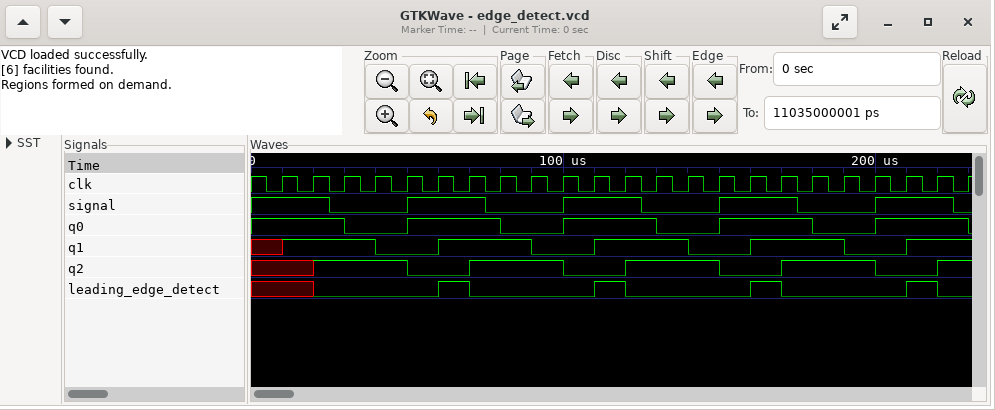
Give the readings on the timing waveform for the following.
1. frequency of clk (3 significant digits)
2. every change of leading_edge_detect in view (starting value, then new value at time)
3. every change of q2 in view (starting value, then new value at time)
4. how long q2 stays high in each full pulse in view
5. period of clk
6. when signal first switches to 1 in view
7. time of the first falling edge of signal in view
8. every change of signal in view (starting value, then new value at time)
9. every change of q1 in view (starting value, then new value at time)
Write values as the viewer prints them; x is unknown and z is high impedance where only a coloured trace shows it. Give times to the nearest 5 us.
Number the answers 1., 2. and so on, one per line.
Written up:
1. 100 kHz
2. x, 0 at 20 us, 1 at 60 us, 0 at 70 us, 1 at 110 us, 0 at 120 us, 1 at 160 us, 0 at 170 us, 1 at 210 us, 0 at 220 us
3. x, 1 at 20 us, 0 at 50 us, 1 at 70 us, 0 at 100 us, 1 at 120 us, 0 at 150 us, 1 at 170 us, 0 at 200 us, 1 at 220 us
4. 30 us, 30 us, 30 us
5. 10 us
6. 50 us
7. 25 us
8. 1, 0 at 25 us, 1 at 50 us, 0 at 75 us, 1 at 100 us, 0 at 125 us, 1 at 150 us, 0 at 175 us, 1 at 200 us, 0 at 225 us
9. x, 1 at 10 us, 0 at 40 us, 1 at 60 us, 0 at 90 us, 1 at 110 us, 0 at 140 us, 1 at 160 us, 0 at 190 us, 1 at 210 us
